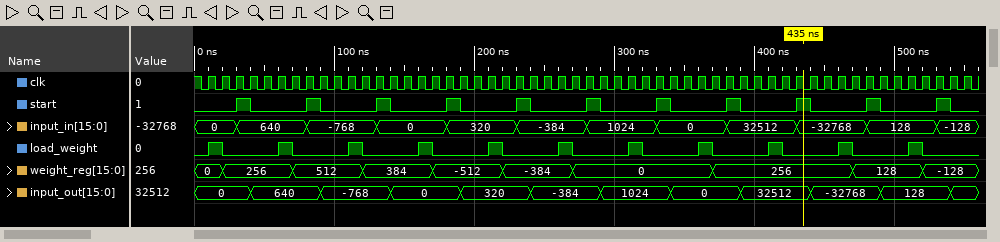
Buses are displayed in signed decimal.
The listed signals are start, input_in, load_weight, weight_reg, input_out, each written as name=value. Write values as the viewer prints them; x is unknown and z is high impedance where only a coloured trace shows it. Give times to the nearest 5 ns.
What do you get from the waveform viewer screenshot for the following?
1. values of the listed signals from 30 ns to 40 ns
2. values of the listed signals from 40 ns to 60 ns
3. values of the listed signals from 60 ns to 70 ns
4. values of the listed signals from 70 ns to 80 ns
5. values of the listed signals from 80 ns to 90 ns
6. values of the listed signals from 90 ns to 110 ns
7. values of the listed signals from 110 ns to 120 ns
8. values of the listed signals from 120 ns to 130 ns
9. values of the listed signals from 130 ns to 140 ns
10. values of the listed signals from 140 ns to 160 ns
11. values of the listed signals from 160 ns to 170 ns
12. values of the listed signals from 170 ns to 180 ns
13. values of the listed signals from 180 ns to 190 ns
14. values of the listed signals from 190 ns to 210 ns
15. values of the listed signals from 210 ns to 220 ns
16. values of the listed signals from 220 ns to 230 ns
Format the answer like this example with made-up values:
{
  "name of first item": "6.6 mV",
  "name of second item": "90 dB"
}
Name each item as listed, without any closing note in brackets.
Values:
{
  "values of the listed signals from 30 ns to 40 ns": "start=1, input_in=640, load_weight=0, weight_reg=256, input_out=0",
  "values of the listed signals from 40 ns to 60 ns": "start=0, input_in=640, load_weight=0, weight_reg=256, input_out=640",
  "values of the listed signals from 60 ns to 70 ns": "start=0, input_in=640, load_weight=1, weight_reg=256, input_out=640",
  "values of the listed signals from 70 ns to 80 ns": "start=0, input_in=640, load_weight=0, weight_reg=512, input_out=640",
  "values of the listed signals from 80 ns to 90 ns": "start=1, input_in=-768, load_weight=0, weight_reg=512, input_out=640",
  "values of the listed signals from 90 ns to 110 ns": "start=0, input_in=-768, load_weight=0, weight_reg=512, input_out=-768",
  "values of the listed signals from 110 ns to 120 ns": "start=0, input_in=-768, load_weight=1, weight_reg=512, input_out=-768",
  "values of the listed signals from 120 ns to 130 ns": "start=0, input_in=-768, load_weight=0, weight_reg=384, input_out=-768",
  "values of the listed signals from 130 ns to 140 ns": "start=1, input_in=0, load_weight=0, weight_reg=384, input_out=-768",
  "values of the listed signals from 140 ns to 160 ns": "start=0, input_in=0, load_weight=0, weight_reg=384, input_out=0",
  "values of the listed signals from 160 ns to 170 ns": "start=0, input_in=0, load_weight=1, weight_reg=384, input_out=0",
  "values of the listed signals from 170 ns to 180 ns": "start=0, input_in=0, load_weight=0, weight_reg=-512, input_out=0",
  "values of the listed signals from 180 ns to 190 ns": "start=1, input_in=320, load_weight=0, weight_reg=-512, input_out=0",
  "values of the listed signals from 190 ns to 210 ns": "start=0, input_in=320, load_weight=0, weight_reg=-512, input_out=320",
  "values of the listed signals from 210 ns to 220 ns": "start=0, input_in=320, load_weight=1, weight_reg=-512, input_out=320",
  "values of the listed signals from 220 ns to 230 ns": "start=0, input_in=320, load_weight=0, weight_reg=-384, input_out=320"
}
